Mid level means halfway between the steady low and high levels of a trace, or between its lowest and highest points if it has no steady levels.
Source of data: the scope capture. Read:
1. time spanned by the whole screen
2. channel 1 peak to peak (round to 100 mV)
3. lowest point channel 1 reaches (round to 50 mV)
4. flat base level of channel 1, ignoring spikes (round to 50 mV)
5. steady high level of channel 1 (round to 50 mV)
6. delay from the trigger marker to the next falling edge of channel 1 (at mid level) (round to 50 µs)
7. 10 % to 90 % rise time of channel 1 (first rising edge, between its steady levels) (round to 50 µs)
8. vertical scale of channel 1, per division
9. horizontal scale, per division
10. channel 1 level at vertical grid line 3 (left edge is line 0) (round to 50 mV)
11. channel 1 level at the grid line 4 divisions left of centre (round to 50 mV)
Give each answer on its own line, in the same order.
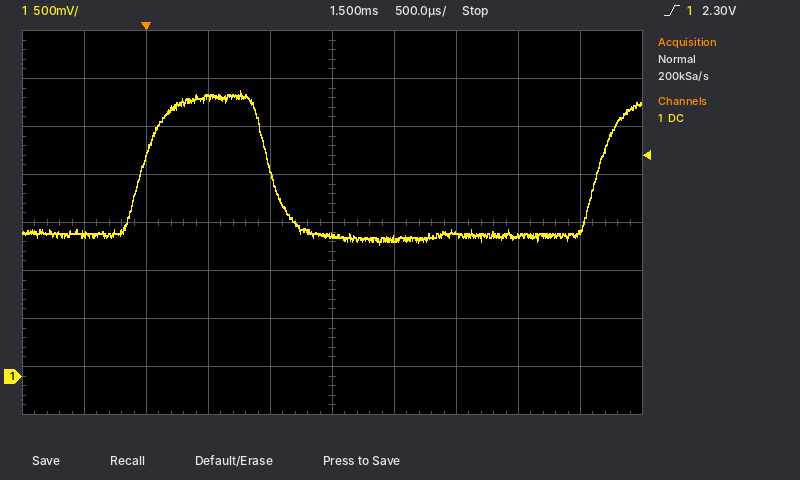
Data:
5 ms
1.60 V
1.35 V
1.45 V
2.90 V
1.00 ms
350 µs
500 mV
500 µs
2.90 V
1.50 V
